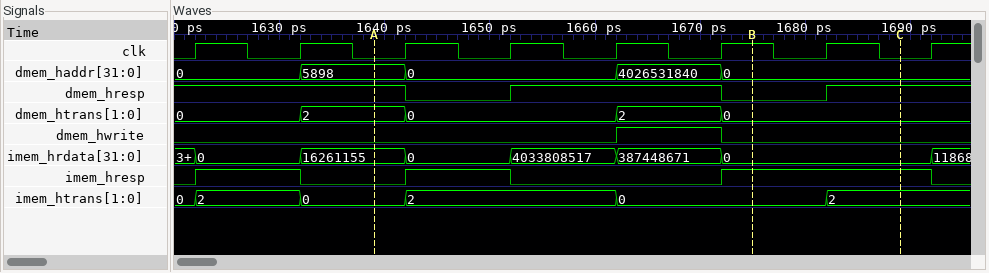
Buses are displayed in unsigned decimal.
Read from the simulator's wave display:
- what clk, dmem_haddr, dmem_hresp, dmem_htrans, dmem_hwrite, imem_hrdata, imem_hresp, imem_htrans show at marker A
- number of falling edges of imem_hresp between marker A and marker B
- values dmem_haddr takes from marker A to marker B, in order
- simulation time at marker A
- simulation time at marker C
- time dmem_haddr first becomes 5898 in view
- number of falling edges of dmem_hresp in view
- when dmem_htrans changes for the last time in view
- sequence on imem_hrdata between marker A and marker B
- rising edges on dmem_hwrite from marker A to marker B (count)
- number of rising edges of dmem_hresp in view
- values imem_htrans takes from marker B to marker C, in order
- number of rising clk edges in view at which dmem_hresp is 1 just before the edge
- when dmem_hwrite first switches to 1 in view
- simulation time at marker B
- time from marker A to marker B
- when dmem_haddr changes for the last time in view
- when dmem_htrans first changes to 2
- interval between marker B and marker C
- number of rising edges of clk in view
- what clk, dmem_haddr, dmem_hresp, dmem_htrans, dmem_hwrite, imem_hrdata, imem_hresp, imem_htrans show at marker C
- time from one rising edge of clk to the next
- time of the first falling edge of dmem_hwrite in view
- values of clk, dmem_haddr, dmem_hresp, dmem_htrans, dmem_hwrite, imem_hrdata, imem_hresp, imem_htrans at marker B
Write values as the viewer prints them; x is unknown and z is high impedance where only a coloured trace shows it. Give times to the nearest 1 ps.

clk=0, dmem_haddr=5898, dmem_hresp=1, dmem_htrans=2, dmem_hwrite=0, imem_hrdata=16261155, imem_hresp=0, imem_htrans=0
1
5898, 0, 4026531840, 0
1639 ps
1689 ps
1632 ps
2
1672 ps
16261155, 0, 4033808517, 387448671, 0
1
2
0, 2
6
1662 ps
1675 ps
36 ps
1672 ps
1632 ps
14 ps
8
clk=0, dmem_haddr=0, dmem_hresp=1, dmem_htrans=0, dmem_hwrite=0, imem_hrdata=0, imem_hresp=1, imem_htrans=2
10 ps
1672 ps
clk=1, dmem_haddr=0, dmem_hresp=0, dmem_htrans=0, dmem_hwrite=0, imem_hrdata=0, imem_hresp=1, imem_htrans=0
